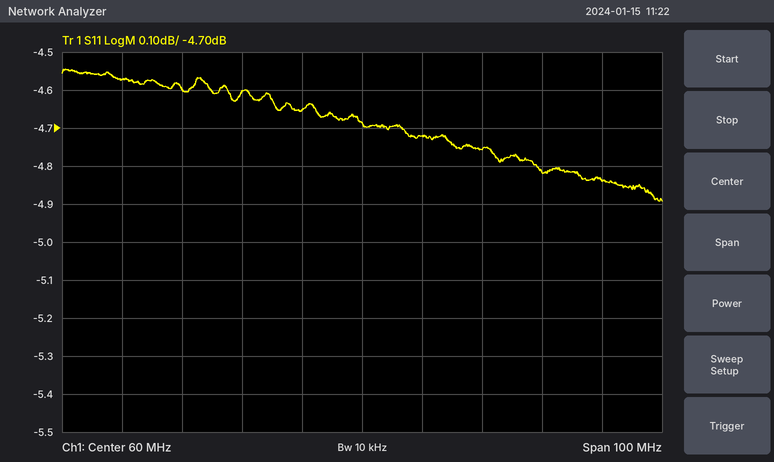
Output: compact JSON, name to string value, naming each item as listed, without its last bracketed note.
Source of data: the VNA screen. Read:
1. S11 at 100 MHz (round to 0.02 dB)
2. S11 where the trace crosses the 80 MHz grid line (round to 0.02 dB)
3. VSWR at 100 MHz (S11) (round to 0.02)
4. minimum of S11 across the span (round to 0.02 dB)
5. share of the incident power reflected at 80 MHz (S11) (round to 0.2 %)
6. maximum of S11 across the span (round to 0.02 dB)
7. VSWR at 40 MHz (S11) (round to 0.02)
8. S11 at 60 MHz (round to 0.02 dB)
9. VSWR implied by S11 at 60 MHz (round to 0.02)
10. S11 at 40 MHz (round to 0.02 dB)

{"S11 at 100 MHz": "-4.84 dB", "S11 where the trace crosses the 80 MHz grid line": "-4.76 dB", "VSWR at 100 MHz (S11)": "3.68", "minimum of S11 across the span": "-4.90 dB", "share of the incident power reflected at 80 MHz (S11)": "33.4 %", "maximum of S11 across the span": "-4.54 dB", "VSWR at 40 MHz (S11)": "3.86", "S11 at 60 MHz": "-4.68 dB", "VSWR implied by S11 at 60 MHz": "3.80", "S11 at 40 MHz": "-4.60 dB"}
